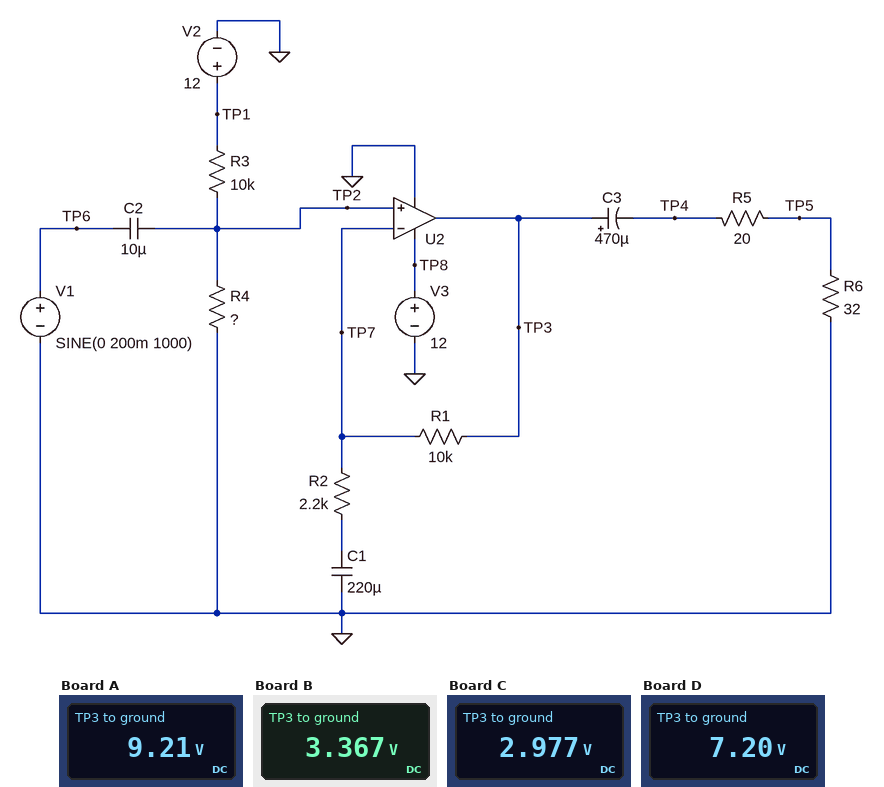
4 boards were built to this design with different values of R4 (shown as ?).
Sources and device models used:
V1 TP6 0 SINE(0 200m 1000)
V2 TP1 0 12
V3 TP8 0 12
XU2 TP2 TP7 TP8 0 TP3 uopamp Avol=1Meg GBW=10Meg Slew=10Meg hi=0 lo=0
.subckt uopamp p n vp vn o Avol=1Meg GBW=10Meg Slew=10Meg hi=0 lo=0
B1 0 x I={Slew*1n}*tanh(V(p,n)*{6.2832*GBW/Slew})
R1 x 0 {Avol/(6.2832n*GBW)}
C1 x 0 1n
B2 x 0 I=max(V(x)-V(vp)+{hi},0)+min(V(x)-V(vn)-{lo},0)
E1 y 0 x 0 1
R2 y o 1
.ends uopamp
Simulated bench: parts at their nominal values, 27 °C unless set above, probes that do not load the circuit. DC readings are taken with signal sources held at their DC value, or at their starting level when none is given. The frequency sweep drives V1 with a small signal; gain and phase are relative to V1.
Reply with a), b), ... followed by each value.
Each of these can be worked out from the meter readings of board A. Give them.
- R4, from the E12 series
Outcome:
a) 33 kΩ
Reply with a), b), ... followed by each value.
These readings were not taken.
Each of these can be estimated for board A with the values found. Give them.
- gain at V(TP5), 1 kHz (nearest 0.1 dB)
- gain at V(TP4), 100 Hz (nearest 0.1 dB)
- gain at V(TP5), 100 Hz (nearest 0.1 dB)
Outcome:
a) 10.7 dB
b) 14.9 dB
c) 10.6 dB
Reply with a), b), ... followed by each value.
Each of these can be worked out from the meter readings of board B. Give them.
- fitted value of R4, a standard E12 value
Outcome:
a) 3.9 kΩ
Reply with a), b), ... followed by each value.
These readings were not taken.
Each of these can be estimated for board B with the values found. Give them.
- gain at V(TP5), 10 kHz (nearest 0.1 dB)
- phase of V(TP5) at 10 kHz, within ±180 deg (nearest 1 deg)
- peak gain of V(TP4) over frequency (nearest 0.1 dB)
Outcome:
a) 10.7 dB
b) 0 deg
c) 14.9 dB
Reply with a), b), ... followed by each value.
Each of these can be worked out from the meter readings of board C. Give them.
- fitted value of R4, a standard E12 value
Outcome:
a) 3.3 kΩ
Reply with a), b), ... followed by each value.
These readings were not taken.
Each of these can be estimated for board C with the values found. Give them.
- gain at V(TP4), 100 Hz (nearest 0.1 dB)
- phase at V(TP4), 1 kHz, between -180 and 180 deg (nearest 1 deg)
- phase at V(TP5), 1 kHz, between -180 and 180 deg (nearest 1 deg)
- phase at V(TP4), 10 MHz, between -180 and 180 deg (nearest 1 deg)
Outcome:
a) 14.8 dB
b) 1 deg
c) 1 deg
d) -80 deg
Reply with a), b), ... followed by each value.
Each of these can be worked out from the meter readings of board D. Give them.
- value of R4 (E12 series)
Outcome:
a) 15 kΩ
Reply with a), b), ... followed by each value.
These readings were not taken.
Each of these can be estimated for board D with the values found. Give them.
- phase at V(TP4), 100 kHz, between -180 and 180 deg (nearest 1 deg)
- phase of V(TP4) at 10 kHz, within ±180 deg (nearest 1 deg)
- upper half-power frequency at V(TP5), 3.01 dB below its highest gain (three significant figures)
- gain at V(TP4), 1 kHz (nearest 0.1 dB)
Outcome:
a) -3 deg
b) 0 deg
c) 1.77 MHz
d) 14.9 dB
